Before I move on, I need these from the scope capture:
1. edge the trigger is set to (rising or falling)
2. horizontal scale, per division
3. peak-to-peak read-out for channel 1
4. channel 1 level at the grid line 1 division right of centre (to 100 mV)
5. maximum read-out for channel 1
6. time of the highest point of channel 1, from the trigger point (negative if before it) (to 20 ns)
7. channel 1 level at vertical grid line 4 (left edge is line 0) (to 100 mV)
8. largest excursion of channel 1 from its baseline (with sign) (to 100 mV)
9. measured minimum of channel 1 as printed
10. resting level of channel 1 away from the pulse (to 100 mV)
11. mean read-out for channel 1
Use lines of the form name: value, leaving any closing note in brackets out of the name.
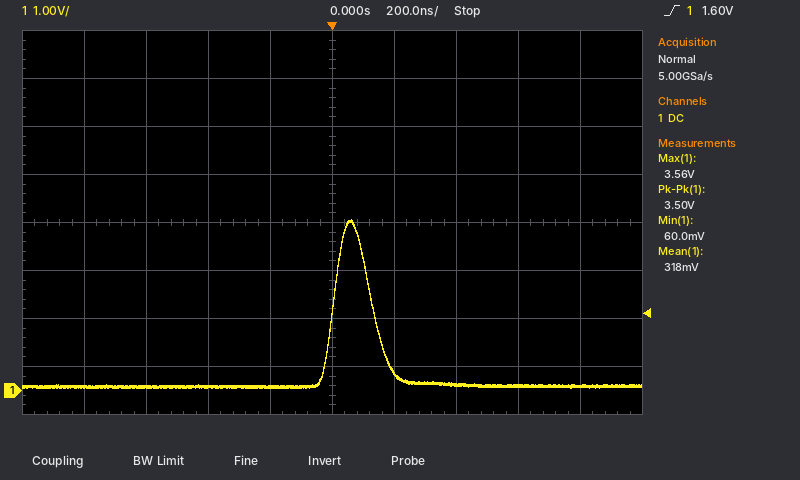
edge the trigger is set to: rising
horizontal scale, per division: 200 ns
peak-to-peak read-out for channel 1: 3.50 V
channel 1 level at the grid line 1 division right of centre: 400 mV
maximum read-out for channel 1: 3.56 V
time of the highest point of channel 1, from the trigger point (negative if before it): +60 ns
channel 1 level at vertical grid line 4 (left edge is line 0): 100 mV
largest excursion of channel 1 from its baseline (with sign): +3.5 V
measured minimum of channel 1 as printed: 60.0 mV
resting level of channel 1 away from the pulse: 100 mV
mean read-out for channel 1: 318 mV
